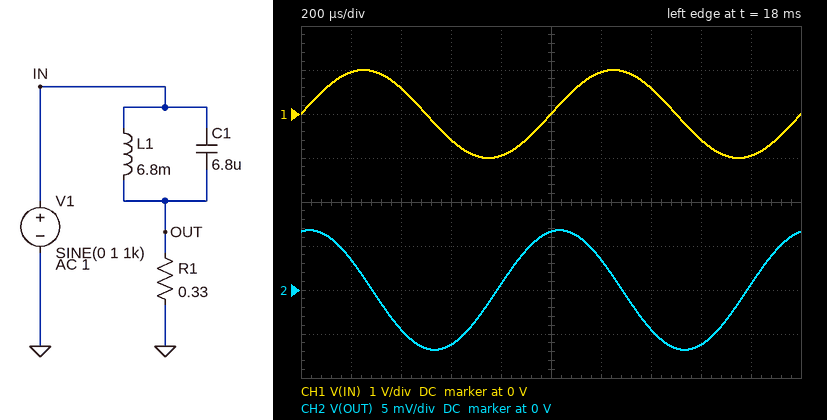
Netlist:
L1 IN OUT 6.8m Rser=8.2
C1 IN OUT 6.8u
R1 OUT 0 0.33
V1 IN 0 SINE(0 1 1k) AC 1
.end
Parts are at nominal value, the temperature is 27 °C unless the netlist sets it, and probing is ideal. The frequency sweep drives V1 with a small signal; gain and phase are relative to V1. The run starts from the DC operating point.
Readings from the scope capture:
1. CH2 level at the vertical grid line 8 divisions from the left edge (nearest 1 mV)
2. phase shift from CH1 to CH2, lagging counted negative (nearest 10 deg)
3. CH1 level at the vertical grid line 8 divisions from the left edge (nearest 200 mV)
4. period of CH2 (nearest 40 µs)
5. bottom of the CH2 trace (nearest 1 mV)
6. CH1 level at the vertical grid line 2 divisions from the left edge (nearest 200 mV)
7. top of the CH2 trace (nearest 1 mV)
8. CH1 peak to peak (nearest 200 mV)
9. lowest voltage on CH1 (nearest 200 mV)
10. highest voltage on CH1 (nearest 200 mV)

-6 mV
80 deg
-600 mV
1.00 ms
-7 mV
600 mV
7 mV
2.0 V
-1.0 V
1.0 V
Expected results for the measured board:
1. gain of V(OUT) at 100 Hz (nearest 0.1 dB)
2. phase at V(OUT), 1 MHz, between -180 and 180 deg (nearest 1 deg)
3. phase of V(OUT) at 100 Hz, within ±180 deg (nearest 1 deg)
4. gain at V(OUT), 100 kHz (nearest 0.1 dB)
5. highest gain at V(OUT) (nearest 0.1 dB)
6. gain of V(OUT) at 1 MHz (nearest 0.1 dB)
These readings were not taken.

-29.4 dB
4 deg
-25 deg
-1.8 dB
0 dB
0 dB
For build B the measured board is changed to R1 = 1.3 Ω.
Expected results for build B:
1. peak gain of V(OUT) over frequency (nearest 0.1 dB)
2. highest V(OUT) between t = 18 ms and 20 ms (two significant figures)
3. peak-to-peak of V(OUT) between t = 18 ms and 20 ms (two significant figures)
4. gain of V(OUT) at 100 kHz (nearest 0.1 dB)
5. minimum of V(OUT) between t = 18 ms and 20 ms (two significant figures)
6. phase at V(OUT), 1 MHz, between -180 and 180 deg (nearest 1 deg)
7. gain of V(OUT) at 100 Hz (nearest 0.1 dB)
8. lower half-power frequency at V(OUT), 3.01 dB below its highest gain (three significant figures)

0 dB
27 mV
53 mV
-0.1 dB
-27 mV
1 deg
-18.2 dB
18.0 kHz
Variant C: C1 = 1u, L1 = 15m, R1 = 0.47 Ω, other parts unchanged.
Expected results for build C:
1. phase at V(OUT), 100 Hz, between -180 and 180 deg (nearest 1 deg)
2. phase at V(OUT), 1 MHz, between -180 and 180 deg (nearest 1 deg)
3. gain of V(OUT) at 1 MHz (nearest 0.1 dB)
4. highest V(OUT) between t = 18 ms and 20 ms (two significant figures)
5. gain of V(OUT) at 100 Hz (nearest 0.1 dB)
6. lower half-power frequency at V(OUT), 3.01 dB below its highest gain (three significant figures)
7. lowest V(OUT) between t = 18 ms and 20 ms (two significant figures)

-47 deg
19 deg
-0.5 dB
2.0 mV
-28.8 dB
339 kHz
-2.0 mV
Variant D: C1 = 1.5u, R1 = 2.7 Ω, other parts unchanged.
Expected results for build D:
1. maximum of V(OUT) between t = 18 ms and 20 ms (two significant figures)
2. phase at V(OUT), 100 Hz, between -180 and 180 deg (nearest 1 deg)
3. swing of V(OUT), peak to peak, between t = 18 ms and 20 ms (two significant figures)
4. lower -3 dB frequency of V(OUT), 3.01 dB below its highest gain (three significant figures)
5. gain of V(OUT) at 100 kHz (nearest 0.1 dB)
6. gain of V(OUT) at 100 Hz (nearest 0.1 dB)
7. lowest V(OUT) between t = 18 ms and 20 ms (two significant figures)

37 mV
-21 deg
74 mV
39.4 kHz
-0.6 dB
-12.8 dB
-37 mV
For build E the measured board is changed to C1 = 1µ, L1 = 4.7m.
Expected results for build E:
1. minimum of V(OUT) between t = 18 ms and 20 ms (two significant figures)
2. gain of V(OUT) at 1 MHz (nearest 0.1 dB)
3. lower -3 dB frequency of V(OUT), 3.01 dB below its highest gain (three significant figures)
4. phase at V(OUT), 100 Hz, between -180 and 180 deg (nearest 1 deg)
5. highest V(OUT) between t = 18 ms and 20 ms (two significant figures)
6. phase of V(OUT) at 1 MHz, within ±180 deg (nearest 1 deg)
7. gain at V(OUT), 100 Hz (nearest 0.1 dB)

-8.8 mV
-0.9 dB
482 kHz
-19 deg
8.8 mV
26 deg
-28.8 dB
